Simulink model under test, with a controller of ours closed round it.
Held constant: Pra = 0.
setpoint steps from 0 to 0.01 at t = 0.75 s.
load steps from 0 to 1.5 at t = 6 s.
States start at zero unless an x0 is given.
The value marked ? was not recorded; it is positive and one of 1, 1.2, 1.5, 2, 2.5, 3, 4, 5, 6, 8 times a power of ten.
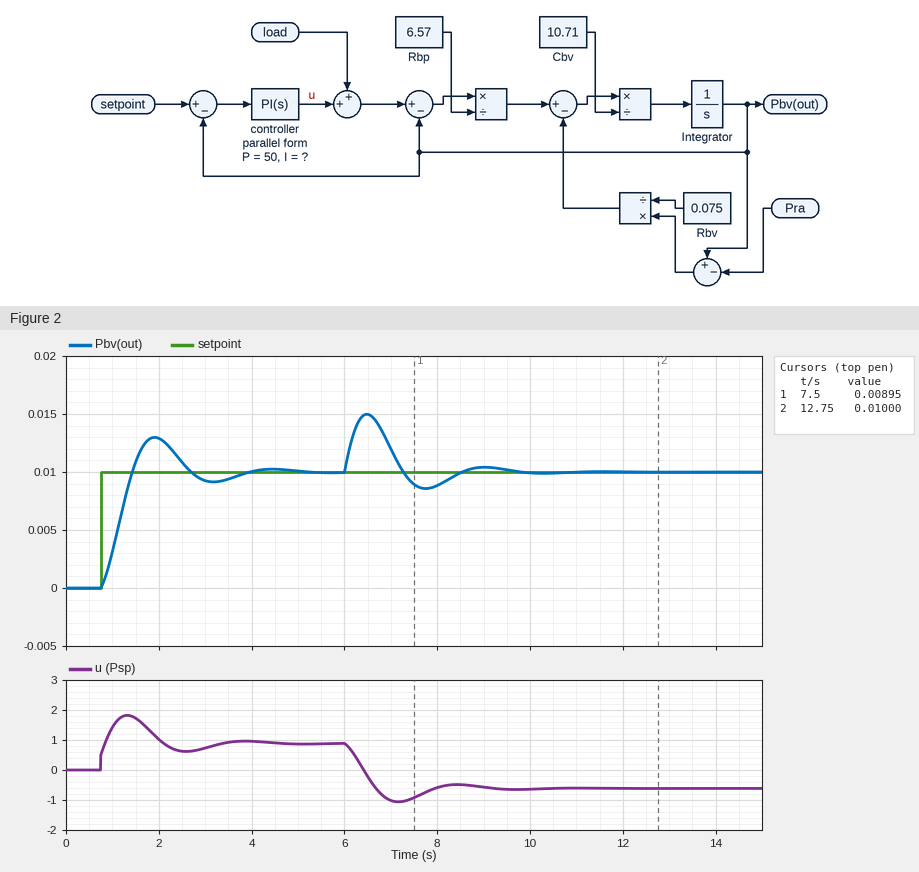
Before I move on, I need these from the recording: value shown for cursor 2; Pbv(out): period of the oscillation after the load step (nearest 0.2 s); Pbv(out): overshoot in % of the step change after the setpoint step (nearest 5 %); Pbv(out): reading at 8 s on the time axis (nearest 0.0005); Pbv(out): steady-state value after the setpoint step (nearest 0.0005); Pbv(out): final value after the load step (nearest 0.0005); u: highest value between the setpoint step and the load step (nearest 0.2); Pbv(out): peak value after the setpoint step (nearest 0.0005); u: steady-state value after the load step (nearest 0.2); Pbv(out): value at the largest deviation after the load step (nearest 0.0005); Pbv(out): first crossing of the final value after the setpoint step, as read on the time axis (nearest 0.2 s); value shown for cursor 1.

0.01000
2.6 s
30 %
0.0090
0.0100
0.0100
1.8
0.0130
-0.6
0.0150
1.4 s
0.00895
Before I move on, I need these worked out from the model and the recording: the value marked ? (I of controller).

500
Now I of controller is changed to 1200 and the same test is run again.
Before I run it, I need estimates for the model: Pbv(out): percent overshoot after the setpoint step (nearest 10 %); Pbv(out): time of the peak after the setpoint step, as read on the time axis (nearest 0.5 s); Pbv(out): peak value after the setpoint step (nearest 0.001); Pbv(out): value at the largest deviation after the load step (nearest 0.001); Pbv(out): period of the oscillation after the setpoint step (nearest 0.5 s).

50 %
1.5 s
0.015
0.014
1.5 s
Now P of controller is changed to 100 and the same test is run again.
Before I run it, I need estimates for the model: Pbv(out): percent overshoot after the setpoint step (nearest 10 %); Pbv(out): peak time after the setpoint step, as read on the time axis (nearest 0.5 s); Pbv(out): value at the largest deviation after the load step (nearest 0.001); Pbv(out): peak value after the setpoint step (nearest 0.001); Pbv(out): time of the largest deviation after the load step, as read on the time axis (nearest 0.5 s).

20 %
2.0 s
0.014
0.012
6.5 s
